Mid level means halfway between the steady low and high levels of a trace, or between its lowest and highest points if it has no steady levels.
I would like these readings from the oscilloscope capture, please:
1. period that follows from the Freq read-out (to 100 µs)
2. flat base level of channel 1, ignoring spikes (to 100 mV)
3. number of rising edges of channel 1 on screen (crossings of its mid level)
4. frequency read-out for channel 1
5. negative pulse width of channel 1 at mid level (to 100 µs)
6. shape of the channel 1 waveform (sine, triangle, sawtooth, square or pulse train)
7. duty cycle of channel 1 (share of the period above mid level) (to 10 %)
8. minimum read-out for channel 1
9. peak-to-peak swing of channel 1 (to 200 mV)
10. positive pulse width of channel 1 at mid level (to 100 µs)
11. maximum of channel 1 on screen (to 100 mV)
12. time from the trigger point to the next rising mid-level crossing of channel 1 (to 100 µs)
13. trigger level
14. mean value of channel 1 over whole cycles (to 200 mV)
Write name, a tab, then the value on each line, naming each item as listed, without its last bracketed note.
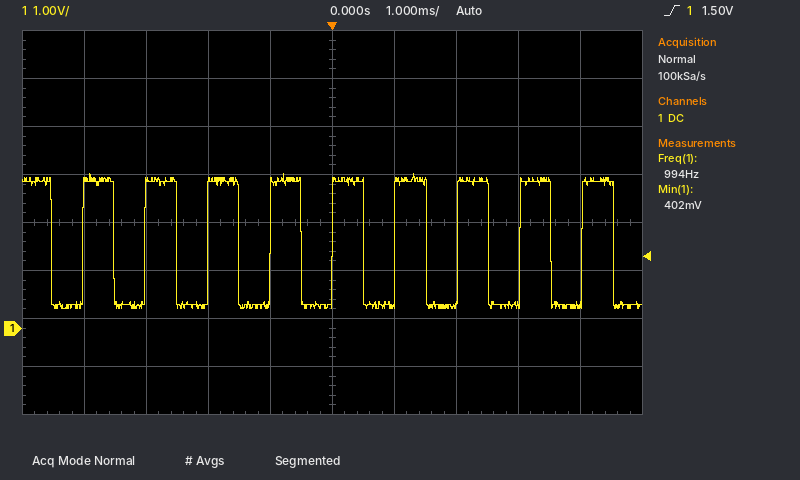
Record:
period that follows from the Freq read-out	1.0 ms
flat base level of channel 1, ignoring spikes	500 mV
number of rising edges of channel 1 on screen	9
frequency read-out for channel 1	994 Hz
negative pulse width of channel 1 at mid level	500 µs
shape of the channel 1 waveform	square
duty cycle of channel 1 (share of the period above mid level)	50 %
minimum read-out for channel 1	402 mV
peak-to-peak swing of channel 1	2.8 V
positive pulse width of channel 1 at mid level	500 µs
maximum of channel 1 on screen	3.2 V
time from the trigger point to the next rising mid-level crossing of channel 1	1.0 ms
trigger level	1.50 V
mean value of channel 1 over whole cycles	1.8 V
